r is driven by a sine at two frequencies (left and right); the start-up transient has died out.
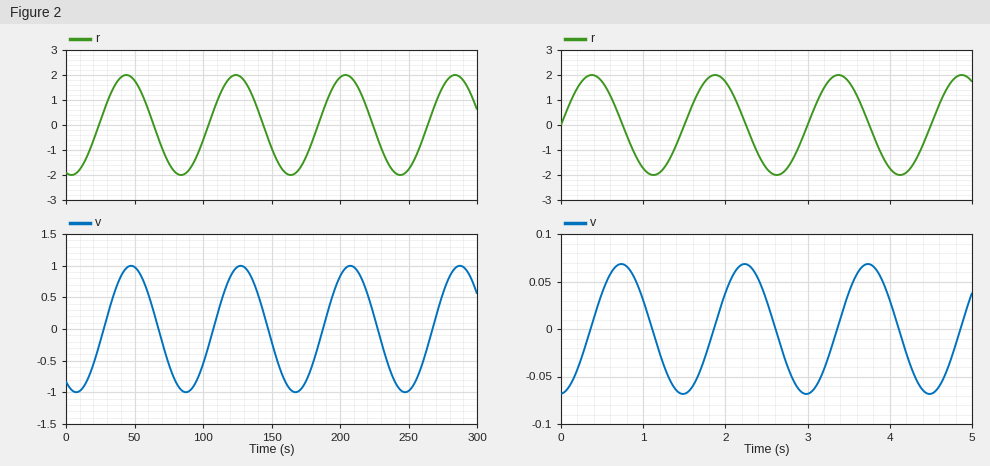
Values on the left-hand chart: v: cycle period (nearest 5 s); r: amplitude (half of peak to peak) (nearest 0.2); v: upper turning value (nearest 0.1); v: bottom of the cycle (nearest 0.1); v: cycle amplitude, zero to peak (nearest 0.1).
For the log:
80 s
2.0
1.0
-1.0
1.0
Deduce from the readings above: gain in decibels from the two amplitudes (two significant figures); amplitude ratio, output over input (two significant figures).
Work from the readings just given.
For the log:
-6.0 dB
0.50
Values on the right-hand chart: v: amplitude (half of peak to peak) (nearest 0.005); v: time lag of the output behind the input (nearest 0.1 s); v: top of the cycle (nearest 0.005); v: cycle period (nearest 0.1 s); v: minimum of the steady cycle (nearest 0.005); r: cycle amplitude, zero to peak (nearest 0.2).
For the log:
0.070
0.4 s
0.070
1.5 s
-0.070
2.0
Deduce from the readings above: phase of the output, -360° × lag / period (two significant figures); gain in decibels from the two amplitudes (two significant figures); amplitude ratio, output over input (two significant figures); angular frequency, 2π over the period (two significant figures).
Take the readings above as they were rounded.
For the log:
-96°
-29 dB
0.035
4.2 rad/s
